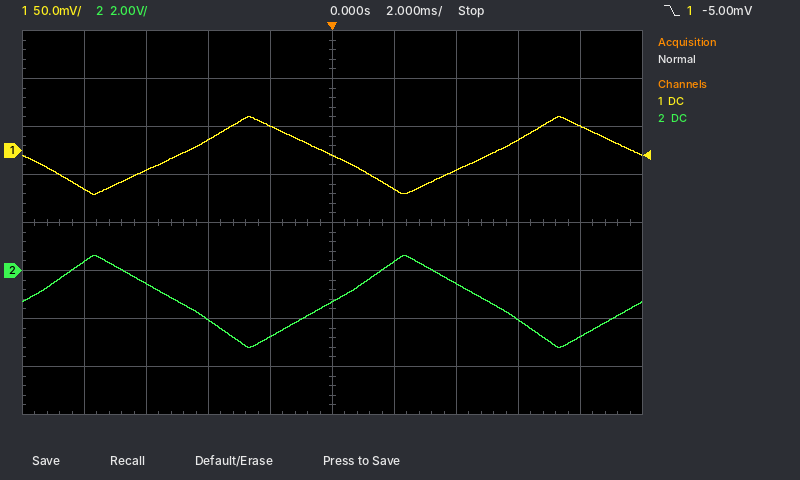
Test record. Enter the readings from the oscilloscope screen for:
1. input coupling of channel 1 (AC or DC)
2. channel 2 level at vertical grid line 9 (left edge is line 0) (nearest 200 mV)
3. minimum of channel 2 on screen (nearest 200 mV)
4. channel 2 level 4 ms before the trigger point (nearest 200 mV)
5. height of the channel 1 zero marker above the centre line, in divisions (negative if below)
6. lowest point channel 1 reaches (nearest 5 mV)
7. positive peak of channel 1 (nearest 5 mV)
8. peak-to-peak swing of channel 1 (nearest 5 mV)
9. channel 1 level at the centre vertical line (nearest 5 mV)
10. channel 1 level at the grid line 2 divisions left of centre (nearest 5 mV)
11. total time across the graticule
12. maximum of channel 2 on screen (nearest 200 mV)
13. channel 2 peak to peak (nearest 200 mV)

DC
-2.8 V
-3.2 V
-2.0 V
+1.5 div
-45 mV
35 mV
80 mV
-5 mV
10 mV
20 ms
600 mV
3.8 V
